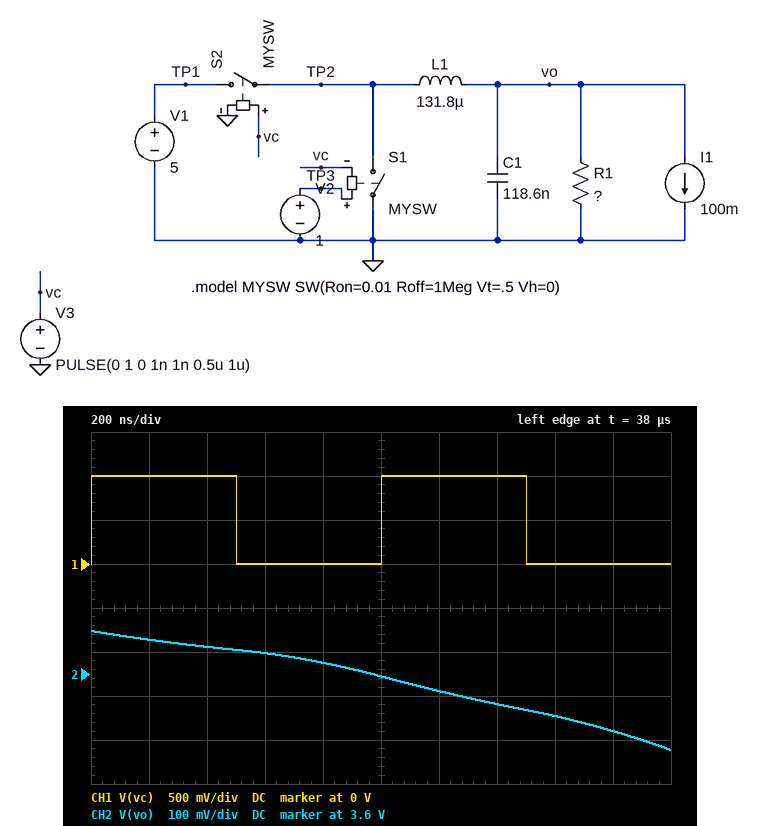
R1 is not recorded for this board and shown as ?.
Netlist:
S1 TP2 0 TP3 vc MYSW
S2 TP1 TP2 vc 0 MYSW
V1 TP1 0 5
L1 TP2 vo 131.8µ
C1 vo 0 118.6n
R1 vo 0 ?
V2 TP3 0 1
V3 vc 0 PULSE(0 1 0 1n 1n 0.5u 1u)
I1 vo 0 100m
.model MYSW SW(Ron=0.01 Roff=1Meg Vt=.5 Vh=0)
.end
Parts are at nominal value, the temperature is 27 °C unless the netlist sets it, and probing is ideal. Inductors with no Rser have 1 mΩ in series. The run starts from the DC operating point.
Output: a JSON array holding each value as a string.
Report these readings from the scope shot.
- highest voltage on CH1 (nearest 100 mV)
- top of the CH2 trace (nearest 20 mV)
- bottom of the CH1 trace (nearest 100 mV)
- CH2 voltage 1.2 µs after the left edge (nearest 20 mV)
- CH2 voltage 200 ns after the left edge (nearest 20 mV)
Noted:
["1.0 V", "3.70 V", "0 V", "3.56 V", "3.68 V"]
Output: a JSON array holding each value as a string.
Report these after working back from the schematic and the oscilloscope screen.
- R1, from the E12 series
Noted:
["220 Ω"]
